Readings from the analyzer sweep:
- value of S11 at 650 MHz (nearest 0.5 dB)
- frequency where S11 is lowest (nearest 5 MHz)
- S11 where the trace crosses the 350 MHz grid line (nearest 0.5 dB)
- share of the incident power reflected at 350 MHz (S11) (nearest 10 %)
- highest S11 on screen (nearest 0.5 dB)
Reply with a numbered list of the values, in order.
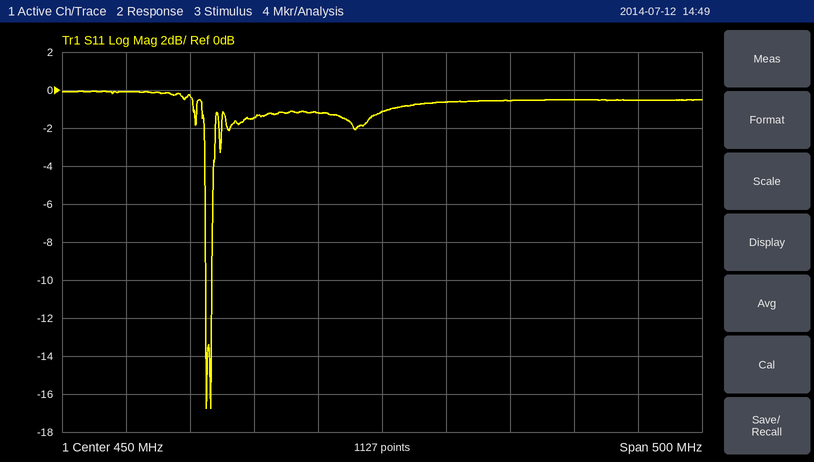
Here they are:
1. -0.5 dB
2. 315 MHz
3. -1.5 dB
4. 70 %
5. 0.0 dB
